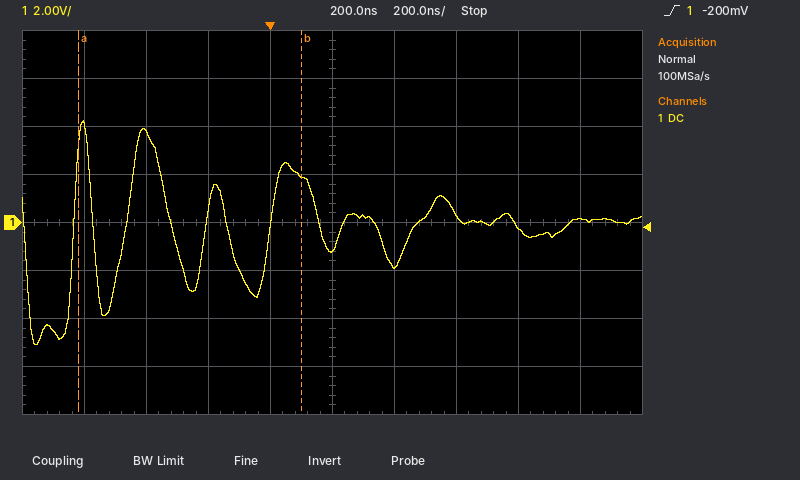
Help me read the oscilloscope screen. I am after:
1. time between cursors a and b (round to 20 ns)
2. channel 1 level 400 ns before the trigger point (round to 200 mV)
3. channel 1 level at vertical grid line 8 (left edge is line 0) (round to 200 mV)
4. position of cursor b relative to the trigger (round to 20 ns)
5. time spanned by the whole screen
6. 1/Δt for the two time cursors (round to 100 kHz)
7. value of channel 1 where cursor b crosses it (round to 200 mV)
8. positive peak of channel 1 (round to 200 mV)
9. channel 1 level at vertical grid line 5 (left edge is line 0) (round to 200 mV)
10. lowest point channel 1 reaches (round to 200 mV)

720 ns
3.8 V
-200 mV
+100 ns
2 µs
1.4 MHz
2.0 V
4.2 V
-1.2 V
-5.0 V
